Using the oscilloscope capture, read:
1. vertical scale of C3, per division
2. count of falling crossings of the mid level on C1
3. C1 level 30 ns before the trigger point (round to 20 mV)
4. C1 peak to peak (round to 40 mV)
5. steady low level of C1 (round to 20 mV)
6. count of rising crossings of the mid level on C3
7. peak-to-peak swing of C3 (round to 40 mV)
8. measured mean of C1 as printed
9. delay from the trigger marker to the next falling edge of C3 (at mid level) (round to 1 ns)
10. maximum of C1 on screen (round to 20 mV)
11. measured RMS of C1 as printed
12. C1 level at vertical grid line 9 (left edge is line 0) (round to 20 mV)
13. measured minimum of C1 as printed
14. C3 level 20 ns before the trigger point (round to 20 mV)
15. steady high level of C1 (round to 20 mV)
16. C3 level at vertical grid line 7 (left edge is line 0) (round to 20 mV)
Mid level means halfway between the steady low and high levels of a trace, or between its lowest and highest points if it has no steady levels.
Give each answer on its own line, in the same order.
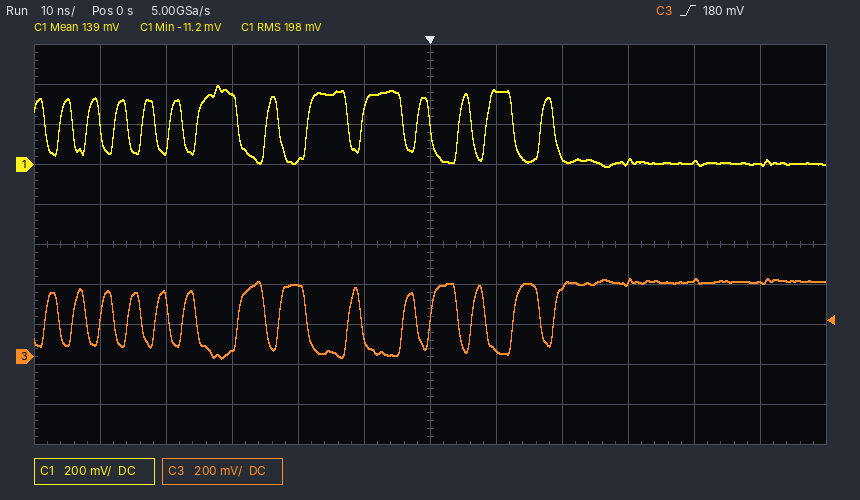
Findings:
200 mV
14
340 mV
400 mV
0 mV
14
400 mV
139 mV
4 ns
400 mV
198 mV
20 mV
-11.2 mV
360 mV
360 mV
40 mV
